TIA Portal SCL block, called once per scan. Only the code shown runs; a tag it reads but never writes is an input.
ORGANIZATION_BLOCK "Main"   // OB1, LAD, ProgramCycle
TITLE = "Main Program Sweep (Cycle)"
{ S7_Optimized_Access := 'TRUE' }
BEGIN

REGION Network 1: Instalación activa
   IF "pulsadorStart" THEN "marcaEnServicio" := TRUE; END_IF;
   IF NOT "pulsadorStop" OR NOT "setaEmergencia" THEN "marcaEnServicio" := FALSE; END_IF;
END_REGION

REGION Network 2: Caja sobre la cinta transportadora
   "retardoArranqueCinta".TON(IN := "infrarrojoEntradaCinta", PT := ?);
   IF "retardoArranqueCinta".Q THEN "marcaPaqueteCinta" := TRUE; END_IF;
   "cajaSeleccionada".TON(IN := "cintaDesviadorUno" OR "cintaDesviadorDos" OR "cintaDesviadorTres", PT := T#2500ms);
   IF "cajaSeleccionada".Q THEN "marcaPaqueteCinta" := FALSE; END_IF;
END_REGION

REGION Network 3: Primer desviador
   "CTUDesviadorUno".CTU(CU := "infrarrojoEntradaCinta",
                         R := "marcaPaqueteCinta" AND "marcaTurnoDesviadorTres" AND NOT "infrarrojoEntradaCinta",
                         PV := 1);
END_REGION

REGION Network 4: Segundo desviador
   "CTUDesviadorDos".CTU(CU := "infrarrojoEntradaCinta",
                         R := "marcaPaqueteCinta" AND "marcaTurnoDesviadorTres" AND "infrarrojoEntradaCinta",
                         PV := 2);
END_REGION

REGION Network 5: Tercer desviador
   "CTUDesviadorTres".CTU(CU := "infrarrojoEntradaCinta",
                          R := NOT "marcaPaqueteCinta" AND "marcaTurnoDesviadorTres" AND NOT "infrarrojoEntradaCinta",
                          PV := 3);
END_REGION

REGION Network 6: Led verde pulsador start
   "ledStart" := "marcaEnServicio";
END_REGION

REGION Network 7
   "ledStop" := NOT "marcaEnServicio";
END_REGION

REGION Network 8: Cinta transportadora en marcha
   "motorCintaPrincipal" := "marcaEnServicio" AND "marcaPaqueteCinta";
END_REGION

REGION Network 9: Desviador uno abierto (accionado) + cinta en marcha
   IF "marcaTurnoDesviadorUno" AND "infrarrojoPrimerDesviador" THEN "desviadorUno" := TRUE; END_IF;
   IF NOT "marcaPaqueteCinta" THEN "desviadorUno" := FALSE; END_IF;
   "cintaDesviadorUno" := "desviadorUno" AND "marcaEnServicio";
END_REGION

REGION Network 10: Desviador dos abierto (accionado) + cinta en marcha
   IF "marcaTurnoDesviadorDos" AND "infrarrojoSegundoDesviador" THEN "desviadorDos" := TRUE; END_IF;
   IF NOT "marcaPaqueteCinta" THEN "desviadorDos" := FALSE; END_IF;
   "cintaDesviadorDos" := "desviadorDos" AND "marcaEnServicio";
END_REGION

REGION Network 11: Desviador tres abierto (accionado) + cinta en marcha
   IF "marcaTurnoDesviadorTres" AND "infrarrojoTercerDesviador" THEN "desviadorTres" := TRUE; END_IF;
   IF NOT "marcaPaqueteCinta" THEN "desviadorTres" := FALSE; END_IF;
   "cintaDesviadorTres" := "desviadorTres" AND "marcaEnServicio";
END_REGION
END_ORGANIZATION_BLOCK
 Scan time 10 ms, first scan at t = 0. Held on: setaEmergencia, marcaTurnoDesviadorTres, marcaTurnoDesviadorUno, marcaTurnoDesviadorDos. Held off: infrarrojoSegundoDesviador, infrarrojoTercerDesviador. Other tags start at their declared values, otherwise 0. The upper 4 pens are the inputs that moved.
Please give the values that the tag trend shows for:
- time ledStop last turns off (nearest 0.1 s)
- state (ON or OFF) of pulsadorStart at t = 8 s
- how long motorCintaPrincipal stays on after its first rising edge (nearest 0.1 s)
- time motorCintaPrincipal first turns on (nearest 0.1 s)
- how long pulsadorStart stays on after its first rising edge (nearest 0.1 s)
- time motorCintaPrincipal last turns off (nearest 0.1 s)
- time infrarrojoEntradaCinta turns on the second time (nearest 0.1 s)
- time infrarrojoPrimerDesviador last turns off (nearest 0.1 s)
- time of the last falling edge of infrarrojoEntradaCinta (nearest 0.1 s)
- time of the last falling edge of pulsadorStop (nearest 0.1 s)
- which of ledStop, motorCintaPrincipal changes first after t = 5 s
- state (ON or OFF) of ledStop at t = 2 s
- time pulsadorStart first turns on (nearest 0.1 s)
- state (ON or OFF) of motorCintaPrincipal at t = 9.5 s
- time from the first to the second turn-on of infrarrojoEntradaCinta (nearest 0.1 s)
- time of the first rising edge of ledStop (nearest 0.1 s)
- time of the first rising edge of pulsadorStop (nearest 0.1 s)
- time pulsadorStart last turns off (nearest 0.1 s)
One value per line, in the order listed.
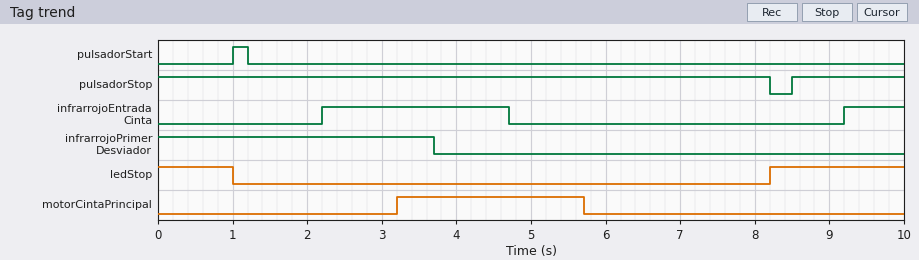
1.0 s
OFF
2.5 s
3.2 s
0.2 s
5.7 s
9.2 s
3.7 s
4.7 s
8.2 s
motorCintaPrincipal
OFF
1.0 s
OFF
7.0 s
8.2 s
8.5 s
1.2 s
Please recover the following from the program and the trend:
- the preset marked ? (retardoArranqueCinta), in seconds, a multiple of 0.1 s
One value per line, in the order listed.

1.0 s
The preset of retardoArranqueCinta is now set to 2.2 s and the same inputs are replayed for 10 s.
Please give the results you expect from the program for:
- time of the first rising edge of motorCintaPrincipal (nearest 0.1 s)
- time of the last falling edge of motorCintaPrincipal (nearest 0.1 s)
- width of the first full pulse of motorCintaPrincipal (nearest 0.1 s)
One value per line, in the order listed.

4.4 s
8.2 s
3.8 s
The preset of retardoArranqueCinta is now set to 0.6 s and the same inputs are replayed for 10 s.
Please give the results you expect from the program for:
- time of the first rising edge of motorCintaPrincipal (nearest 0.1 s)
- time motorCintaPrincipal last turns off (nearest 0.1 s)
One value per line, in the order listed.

2.8 s
5.3 s
